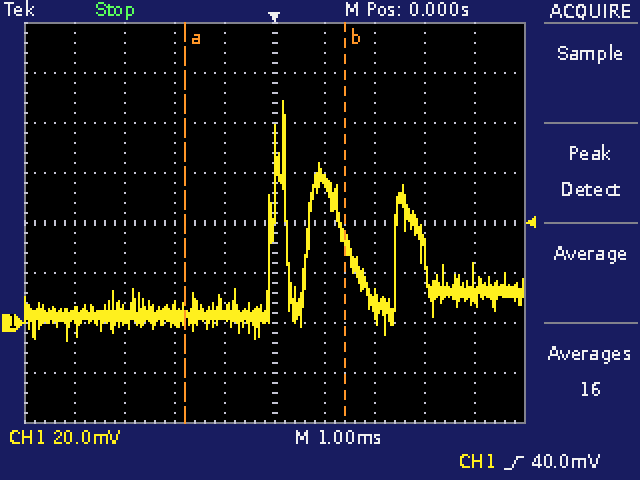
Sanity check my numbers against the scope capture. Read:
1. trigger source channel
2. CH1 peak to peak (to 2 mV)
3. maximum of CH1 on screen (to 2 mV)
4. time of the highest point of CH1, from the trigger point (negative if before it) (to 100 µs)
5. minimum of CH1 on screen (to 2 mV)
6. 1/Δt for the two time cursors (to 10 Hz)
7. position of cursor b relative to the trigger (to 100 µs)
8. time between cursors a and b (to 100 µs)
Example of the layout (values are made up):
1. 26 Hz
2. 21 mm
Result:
1. CH1
2. 96 mV
3. 88 mV
4. +200 µs
5. -8 mV
6. 310 Hz
7. +1.4 ms
8. 3.2 ms
